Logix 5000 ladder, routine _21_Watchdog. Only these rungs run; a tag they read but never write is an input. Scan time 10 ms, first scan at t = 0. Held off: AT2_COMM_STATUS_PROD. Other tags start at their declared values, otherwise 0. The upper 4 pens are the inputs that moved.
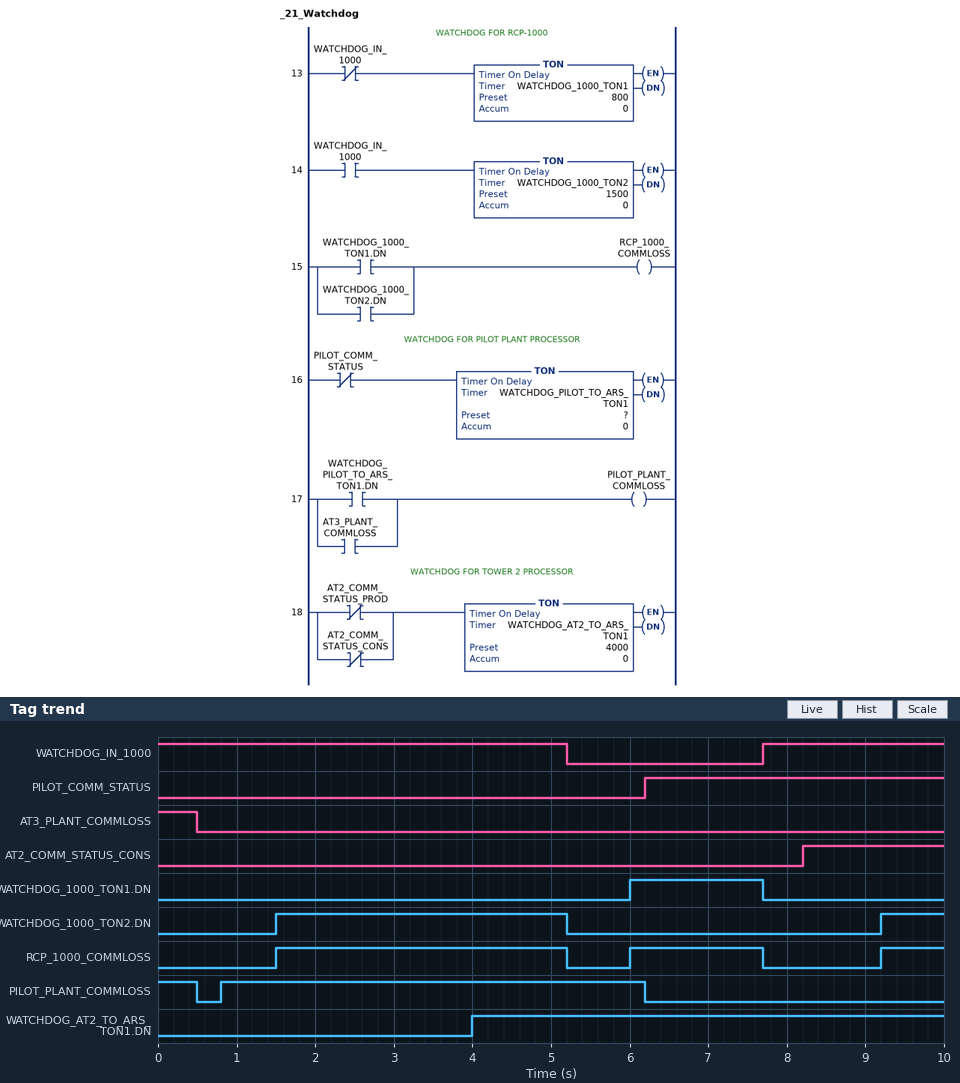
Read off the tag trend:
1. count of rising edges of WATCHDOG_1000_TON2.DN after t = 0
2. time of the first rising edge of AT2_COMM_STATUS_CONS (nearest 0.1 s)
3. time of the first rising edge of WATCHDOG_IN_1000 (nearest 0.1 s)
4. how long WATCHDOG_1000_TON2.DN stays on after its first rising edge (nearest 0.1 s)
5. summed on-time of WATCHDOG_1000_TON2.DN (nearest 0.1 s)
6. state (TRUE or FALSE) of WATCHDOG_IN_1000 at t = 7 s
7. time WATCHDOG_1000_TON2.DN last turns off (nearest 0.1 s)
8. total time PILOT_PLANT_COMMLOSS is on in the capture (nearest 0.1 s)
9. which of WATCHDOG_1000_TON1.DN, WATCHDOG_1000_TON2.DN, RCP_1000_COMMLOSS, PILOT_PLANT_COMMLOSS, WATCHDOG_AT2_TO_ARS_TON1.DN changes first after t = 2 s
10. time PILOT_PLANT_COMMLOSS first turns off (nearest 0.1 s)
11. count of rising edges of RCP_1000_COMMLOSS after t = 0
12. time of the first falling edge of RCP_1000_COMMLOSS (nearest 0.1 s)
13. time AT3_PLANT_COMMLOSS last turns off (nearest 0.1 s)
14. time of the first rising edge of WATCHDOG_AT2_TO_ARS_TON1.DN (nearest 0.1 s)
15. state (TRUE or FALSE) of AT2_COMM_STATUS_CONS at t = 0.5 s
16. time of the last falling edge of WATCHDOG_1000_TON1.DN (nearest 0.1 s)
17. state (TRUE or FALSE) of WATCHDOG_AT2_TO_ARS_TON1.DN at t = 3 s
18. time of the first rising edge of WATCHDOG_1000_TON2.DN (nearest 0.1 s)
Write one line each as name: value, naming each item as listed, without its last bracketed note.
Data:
count of rising edges of WATCHDOG_1000_TON2.DN after t = 0: 2
time of the first rising edge of AT2_COMM_STATUS_CONS: 8.2 s
time of the first rising edge of WATCHDOG_IN_1000: 7.7 s
how long WATCHDOG_1000_TON2.DN stays on after its first rising edge: 3.7 s
summed on-time of WATCHDOG_1000_TON2.DN: 4.5 s
state (TRUE or FALSE) of WATCHDOG_IN_1000 at t = 7 s: FALSE
time WATCHDOG_1000_TON2.DN last turns off: 5.2 s
total time PILOT_PLANT_COMMLOSS is on in the capture: 5.9 s
which of WATCHDOG_1000_TON1.DN, WATCHDOG_1000_TON2.DN, RCP_1000_COMMLOSS, PILOT_PLANT_COMMLOSS, WATCHDOG_AT2_TO_ARS_TON1.DN changes first after t = 2 s: WATCHDOG_AT2_TO_ARS_TON1.DN
time PILOT_PLANT_COMMLOSS first turns off: 0.5 s
count of rising edges of RCP_1000_COMMLOSS after t = 0: 3
time of the first falling edge of RCP_1000_COMMLOSS: 5.2 s
time AT3_PLANT_COMMLOSS last turns off: 0.5 s
time of the first rising edge of WATCHDOG_AT2_TO_ARS_TON1.DN: 4.0 s
state (TRUE or FALSE) of AT2_COMM_STATUS_CONS at t = 0.5 s: FALSE
time of the last falling edge of WATCHDOG_1000_TON1.DN: 7.7 s
state (TRUE or FALSE) of WATCHDOG_AT2_TO_ARS_TON1.DN at t = 3 s: FALSE
time of the first rising edge of WATCHDOG_1000_TON2.DN: 1.5 s
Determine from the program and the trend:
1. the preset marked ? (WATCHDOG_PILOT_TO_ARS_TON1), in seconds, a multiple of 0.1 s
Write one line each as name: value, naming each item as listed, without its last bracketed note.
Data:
the preset marked ? (WATCHDOG_PILOT_TO_ARS_TON1), in seconds, a multiple of 0.1 s: 0.8 s
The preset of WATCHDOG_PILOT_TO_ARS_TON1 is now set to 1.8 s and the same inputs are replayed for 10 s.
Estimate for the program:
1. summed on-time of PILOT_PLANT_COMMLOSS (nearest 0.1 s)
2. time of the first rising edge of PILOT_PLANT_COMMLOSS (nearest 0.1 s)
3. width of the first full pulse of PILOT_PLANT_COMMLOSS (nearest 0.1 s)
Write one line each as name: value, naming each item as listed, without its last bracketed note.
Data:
summed on-time of PILOT_PLANT_COMMLOSS: 4.9 s
time of the first rising edge of PILOT_PLANT_COMMLOSS: 1.8 s
width of the first full pulse of PILOT_PLANT_COMMLOSS: 4.4 s
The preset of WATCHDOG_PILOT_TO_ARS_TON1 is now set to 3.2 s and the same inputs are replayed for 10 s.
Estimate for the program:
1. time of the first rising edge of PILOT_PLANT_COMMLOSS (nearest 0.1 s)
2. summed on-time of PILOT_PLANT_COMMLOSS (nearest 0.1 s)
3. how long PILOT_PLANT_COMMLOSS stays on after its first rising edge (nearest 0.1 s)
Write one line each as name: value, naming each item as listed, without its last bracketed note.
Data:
time of the first rising edge of PILOT_PLANT_COMMLOSS: 3.2 s
summed on-time of PILOT_PLANT_COMMLOSS: 3.5 s
how long PILOT_PLANT_COMMLOSS stays on after its first rising edge: 3.0 s
